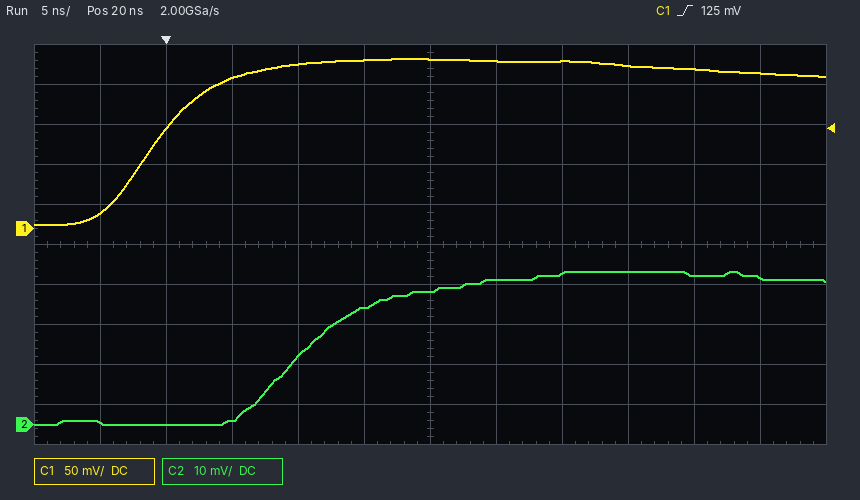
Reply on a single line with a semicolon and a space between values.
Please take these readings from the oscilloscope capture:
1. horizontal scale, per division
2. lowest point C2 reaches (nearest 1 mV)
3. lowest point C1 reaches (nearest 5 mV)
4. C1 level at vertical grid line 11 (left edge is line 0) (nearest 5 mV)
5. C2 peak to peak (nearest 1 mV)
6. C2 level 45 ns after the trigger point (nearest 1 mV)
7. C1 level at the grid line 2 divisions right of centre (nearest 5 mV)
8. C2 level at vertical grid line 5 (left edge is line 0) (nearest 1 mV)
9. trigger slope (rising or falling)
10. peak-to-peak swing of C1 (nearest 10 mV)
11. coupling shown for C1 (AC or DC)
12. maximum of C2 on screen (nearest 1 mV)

5 ns; 0 mV; 5 mV; 195 mV; 38 mV; 37 mV; 210 mV; 29 mV; rising; 210 mV; DC; 38 mV
